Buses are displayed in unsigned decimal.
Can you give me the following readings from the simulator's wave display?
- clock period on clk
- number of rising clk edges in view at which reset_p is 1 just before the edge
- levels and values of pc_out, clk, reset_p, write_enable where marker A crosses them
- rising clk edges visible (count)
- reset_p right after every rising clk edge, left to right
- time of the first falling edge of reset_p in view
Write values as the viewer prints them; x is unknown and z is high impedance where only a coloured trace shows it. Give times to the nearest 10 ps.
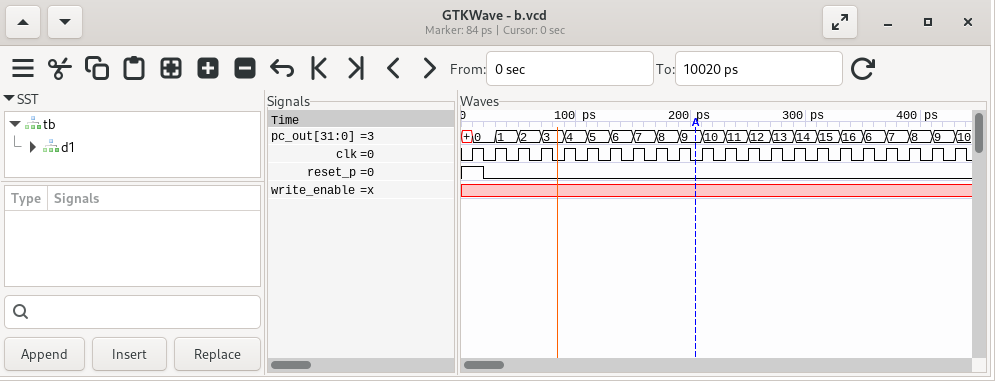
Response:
20 ps
1
pc_out=9, clk=0, reset_p=0, write_enable=x
22
1 0 0 0 0 0 0 0 0 0 0 0 0 0 0 0 0 0 0 0 0 0
20 ps
